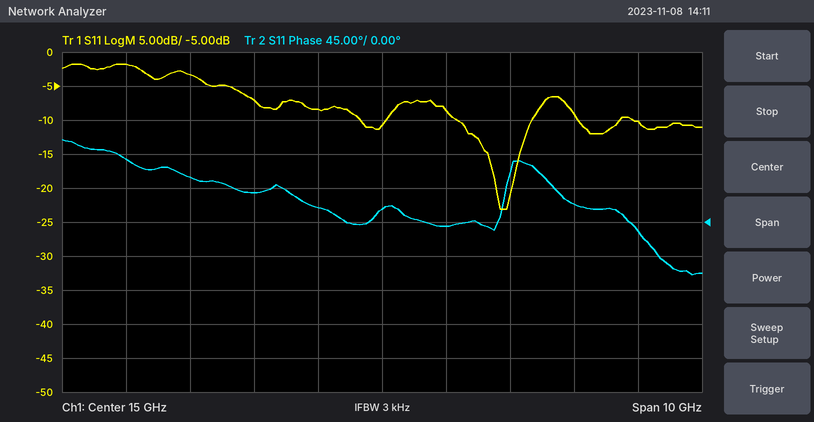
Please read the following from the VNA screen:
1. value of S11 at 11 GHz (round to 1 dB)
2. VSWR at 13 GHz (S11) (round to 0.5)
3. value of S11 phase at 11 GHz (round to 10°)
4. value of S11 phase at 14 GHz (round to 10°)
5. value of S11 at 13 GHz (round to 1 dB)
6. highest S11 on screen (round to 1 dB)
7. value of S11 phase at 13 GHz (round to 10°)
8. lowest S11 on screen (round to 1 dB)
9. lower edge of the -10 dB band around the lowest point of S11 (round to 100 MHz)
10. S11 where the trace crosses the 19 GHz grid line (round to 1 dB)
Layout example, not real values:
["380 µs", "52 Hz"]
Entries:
["-2 dB", "2.5", "80°", "20°", "-7 dB", "-2 dB", "40°", "-23 dB", "16.2 GHz", "-10 dB"]
